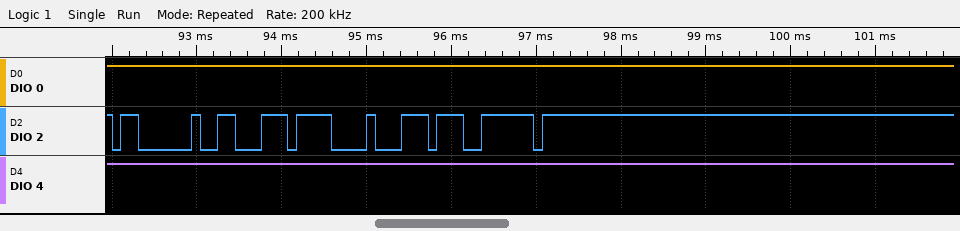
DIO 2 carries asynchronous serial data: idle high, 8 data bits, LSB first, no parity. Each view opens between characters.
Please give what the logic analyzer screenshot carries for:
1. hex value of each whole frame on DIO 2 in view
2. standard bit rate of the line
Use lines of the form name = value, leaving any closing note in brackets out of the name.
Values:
hex value of each whole frame on DIO 2 in view = 03, C6, 0F, DC, 7E
standard bit rate of the line = 9600 baud
